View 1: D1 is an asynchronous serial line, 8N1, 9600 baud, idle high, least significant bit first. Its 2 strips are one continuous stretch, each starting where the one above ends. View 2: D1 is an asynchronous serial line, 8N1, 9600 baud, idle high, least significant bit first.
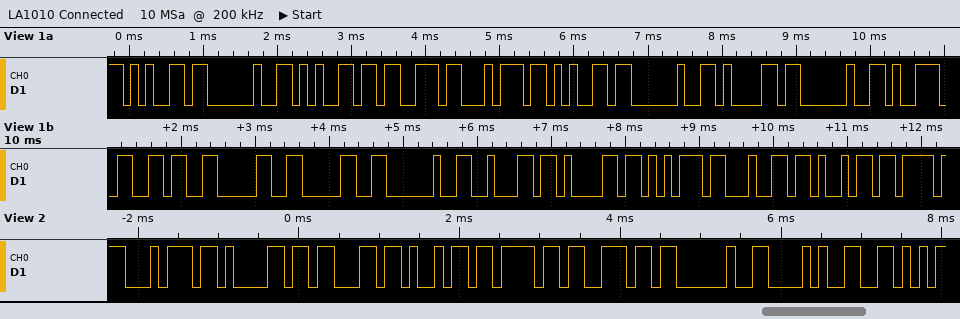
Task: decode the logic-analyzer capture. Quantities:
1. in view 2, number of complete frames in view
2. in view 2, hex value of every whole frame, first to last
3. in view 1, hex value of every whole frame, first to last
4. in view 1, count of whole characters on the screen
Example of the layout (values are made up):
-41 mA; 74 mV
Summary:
9; 74 61 63 69 6F 6E 20 28 56; 65 20 65 73 74 65 20 61 20 39 36 30 30 20 62 61 75 64 69; 19
